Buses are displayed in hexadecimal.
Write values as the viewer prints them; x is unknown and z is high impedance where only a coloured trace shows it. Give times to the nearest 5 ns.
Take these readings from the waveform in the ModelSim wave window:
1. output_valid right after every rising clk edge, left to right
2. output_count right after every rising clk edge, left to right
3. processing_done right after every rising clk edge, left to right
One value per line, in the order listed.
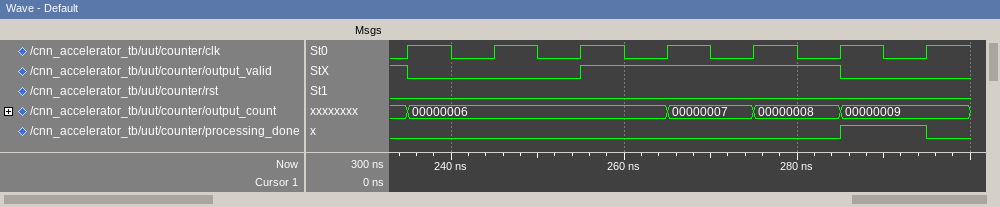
0 0 1 1 1 0 0
00000006, 00000006, 00000006, 00000007, 00000008, 00000009, 00000009
0 0 0 0 0 1 0
